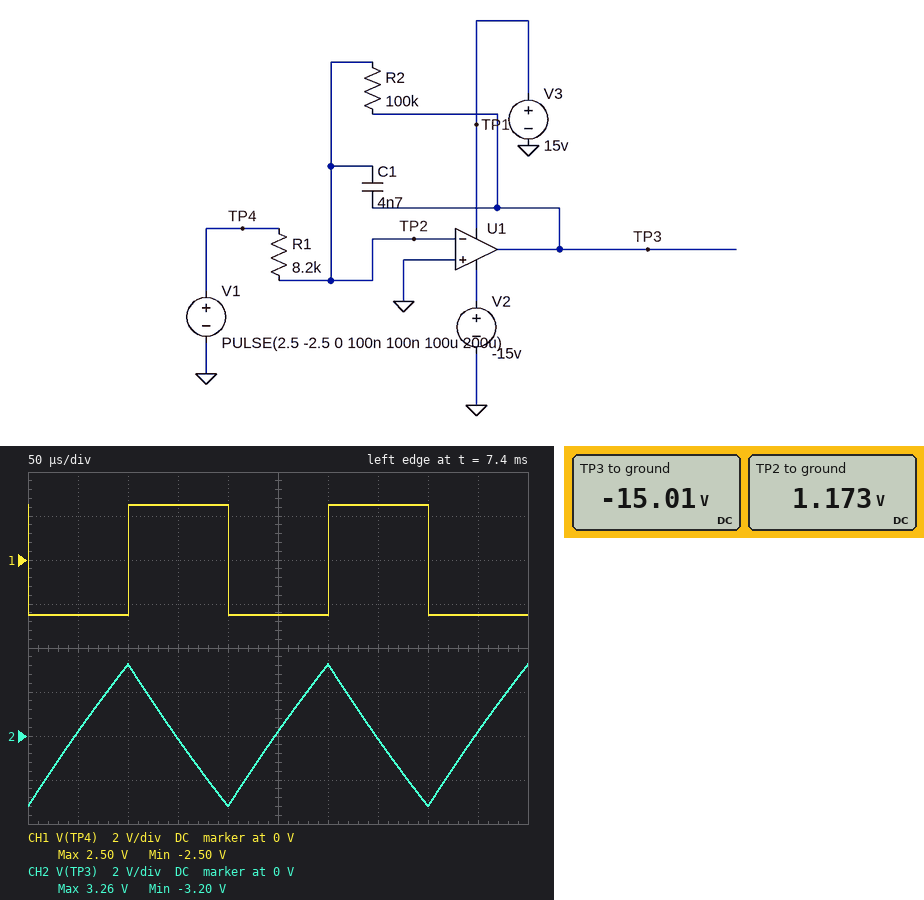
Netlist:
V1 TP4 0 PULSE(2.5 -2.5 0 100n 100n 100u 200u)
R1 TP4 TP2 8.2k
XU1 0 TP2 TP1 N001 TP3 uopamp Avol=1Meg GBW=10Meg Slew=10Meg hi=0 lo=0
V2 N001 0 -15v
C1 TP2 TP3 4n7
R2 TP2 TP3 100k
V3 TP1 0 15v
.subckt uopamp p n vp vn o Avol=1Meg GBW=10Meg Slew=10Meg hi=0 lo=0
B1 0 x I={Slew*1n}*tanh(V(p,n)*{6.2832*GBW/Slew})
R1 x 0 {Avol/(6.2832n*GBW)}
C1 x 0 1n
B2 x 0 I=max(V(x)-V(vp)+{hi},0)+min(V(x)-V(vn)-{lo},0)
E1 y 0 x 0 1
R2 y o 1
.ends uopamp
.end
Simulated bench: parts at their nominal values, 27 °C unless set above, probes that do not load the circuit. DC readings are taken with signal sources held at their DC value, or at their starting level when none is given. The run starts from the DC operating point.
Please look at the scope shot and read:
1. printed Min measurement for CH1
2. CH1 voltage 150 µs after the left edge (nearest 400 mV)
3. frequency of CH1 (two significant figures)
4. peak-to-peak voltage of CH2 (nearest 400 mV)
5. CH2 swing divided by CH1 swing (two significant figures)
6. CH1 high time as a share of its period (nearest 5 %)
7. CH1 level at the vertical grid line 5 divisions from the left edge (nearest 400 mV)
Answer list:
-2.50 V
2.4 V
5.0 kHz
6.4 V
1.3
50 %
-2.4 V
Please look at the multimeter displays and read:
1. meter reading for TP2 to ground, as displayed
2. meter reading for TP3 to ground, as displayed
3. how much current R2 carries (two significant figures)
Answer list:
1.173 V
-15.01 V
160 µA
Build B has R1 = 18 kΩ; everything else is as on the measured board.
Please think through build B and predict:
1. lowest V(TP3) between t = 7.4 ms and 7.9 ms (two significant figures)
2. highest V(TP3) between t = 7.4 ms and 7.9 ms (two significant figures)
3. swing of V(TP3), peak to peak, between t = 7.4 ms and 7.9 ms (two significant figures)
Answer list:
-1.5 V
1.5 V
2.9 V
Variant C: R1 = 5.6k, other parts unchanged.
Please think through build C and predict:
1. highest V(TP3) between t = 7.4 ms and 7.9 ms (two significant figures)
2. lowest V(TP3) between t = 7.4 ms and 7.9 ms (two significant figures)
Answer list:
4.8 V
-4.7 V
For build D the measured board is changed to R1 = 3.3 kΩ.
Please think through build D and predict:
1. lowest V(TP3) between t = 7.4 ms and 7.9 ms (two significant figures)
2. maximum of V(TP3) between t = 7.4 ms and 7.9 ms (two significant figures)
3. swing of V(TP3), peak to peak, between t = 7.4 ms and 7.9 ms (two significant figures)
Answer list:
-7.9 V
8.1 V
16 V
